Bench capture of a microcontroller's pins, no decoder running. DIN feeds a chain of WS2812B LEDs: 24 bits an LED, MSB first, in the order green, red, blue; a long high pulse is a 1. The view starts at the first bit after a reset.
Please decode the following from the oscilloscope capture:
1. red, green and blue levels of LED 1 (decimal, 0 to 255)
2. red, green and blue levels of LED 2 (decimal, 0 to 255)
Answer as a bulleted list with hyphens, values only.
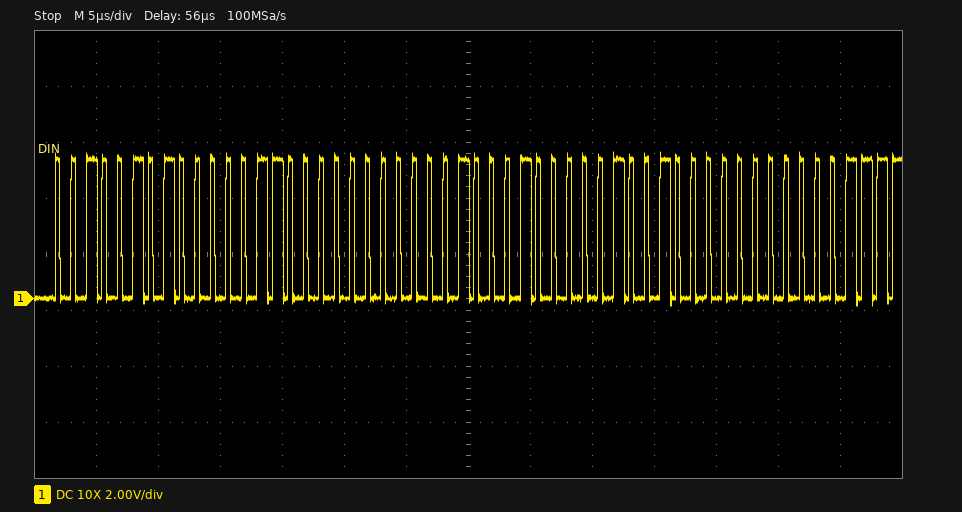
- 6, 37, 0
- 9, 34, 0
